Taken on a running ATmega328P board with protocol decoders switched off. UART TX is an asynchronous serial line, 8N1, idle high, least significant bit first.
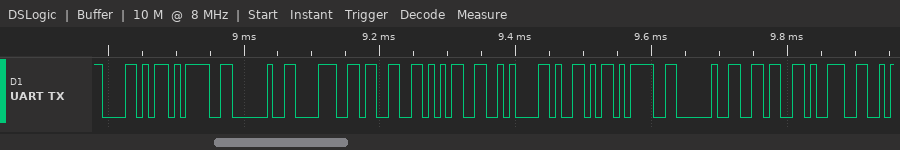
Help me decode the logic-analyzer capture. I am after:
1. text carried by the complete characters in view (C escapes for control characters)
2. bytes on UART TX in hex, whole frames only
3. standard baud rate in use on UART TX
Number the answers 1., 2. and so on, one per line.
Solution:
1. "X= 835\nY= 69"
2. 0x58 0x3D 0x20 0x38 0x33 0x35 0x0A 0x59 0x3D 0x20 0x36 0x39
3. 115200 baud
